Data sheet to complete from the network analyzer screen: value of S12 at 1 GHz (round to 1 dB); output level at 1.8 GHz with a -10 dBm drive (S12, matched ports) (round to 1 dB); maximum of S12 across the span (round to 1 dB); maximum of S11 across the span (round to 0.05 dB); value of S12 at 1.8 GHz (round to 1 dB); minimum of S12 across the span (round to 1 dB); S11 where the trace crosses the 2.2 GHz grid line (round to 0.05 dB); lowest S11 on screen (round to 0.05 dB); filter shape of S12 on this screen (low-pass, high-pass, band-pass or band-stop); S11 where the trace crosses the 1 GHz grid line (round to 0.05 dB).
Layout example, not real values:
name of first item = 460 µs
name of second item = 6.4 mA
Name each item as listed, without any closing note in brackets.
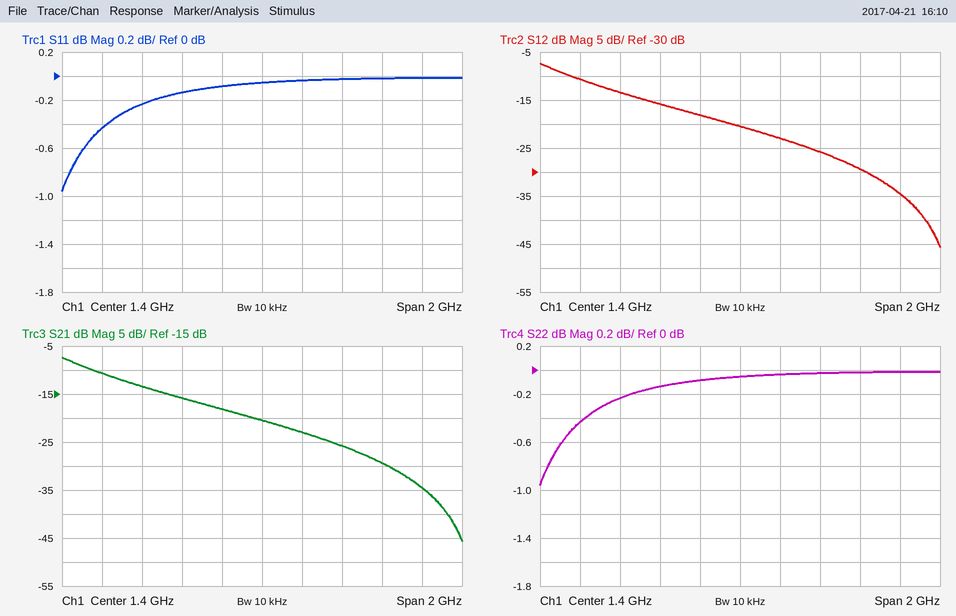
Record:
value of S12 at 1 GHz = -16 dB
output level at 1.8 GHz with a -10 dBm drive (S12, matched ports) = -36 dBm
maximum of S12 across the span = -7 dB
maximum of S11 across the span = 0.00 dB
value of S12 at 1.8 GHz = -26 dB
minimum of S12 across the span = -46 dB
S11 where the trace crosses the 2.2 GHz grid line = 0.00 dB
lowest S11 on screen = -0.95 dB
filter shape of S12 on this screen = low-pass
S11 where the trace crosses the 1 GHz grid line = -0.15 dB
